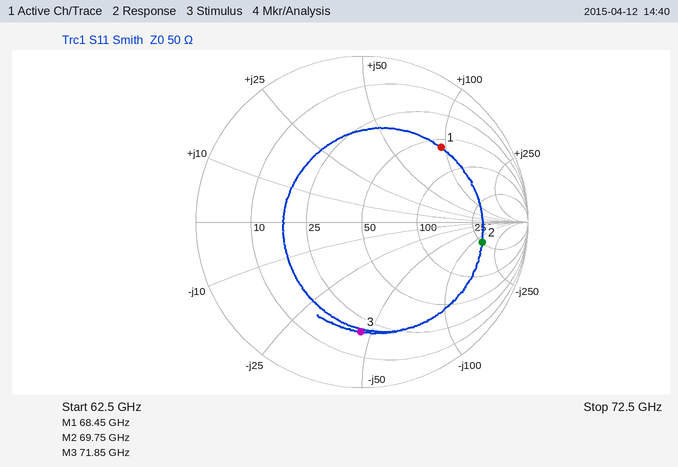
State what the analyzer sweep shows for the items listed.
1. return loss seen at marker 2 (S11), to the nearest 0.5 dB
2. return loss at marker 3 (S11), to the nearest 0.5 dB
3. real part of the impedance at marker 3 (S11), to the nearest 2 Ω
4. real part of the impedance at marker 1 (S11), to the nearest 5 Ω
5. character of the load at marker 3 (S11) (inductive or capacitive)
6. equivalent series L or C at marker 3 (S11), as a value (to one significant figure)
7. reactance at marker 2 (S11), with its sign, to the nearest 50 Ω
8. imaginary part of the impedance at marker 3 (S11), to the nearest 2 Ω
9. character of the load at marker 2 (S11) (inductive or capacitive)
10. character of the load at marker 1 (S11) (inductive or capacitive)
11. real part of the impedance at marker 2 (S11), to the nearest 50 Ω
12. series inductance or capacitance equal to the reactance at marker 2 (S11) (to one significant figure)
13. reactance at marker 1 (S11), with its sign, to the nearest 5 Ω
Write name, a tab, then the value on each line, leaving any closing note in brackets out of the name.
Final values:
return loss seen at marker 2 (S11), to the nearest 0.5 dB	2.5 dB
return loss at marker 3 (S11), to the nearest 0.5 dB	3.5 dB
real part of the impedance at marker 3 (S11), to the nearest 2 Ω	20 Ω
real part of the impedance at marker 1 (S11), to the nearest 5 Ω	60 Ω
character of the load at marker 3 (S11)	capacitive
equivalent series L or C at marker 3 (S11), as a value	50 fF
reactance at marker 2 (S11), with its sign, to the nearest 50 Ω	-150 Ω
imaginary part of the impedance at marker 3 (S11), to the nearest 2 Ω	-46 Ω
character of the load at marker 2 (S11)	capacitive
character of the load at marker 1 (S11)	inductive
real part of the impedance at marker 2 (S11), to the nearest 50 Ω	250 Ω
series inductance or capacitance equal to the reactance at marker 2 (S11)	20 fF
reactance at marker 1 (S11), with its sign, to the nearest 5 Ω	+95 Ω
